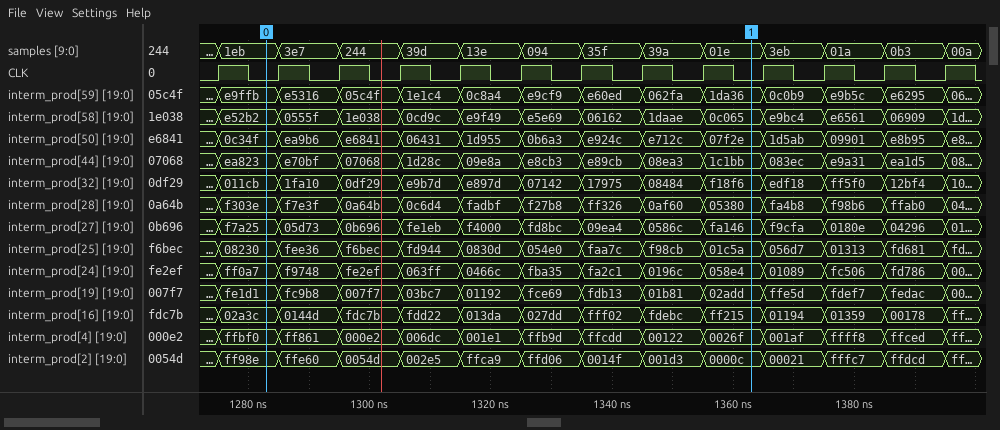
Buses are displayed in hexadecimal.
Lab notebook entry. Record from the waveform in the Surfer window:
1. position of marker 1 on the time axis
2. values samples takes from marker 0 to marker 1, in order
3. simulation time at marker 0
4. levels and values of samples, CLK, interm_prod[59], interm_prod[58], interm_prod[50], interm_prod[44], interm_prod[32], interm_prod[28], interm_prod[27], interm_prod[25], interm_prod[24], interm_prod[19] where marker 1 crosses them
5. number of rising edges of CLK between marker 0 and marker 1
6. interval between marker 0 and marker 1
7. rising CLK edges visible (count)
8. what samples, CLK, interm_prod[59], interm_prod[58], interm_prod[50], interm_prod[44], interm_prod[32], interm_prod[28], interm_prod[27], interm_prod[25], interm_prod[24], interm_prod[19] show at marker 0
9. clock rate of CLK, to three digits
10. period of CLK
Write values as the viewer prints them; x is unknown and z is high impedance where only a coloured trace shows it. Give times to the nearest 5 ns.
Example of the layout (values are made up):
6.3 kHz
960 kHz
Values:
1365 ns
1eb, 3e7, 244, 39d, 13e, 094, 35f, 39a, 01e
1285 ns
samples=01e, CLK=0, interm_prod[59]=1da36, interm_prod[58]=0c065, interm_prod[50]=07f2e, interm_prod[44]=1c1bb, interm_prod[32]=f18f6, interm_prod[28]=05380, interm_prod[27]=fa146, interm_prod[25]=01c5a, interm_prod[24]=058e4, interm_prod[19]=02add
8
80 ns
13
samples=1eb, CLK=0, interm_prod[59]=e9ffb, interm_prod[58]=e52b2, interm_prod[50]=0c34f, interm_prod[44]=ea823, interm_prod[32]=011cb, interm_prod[28]=f303e, interm_prod[27]=f7a25, interm_prod[25]=08230, interm_prod[24]=ff0a7, interm_prod[19]=fe1d1
100 MHz
10 ns
